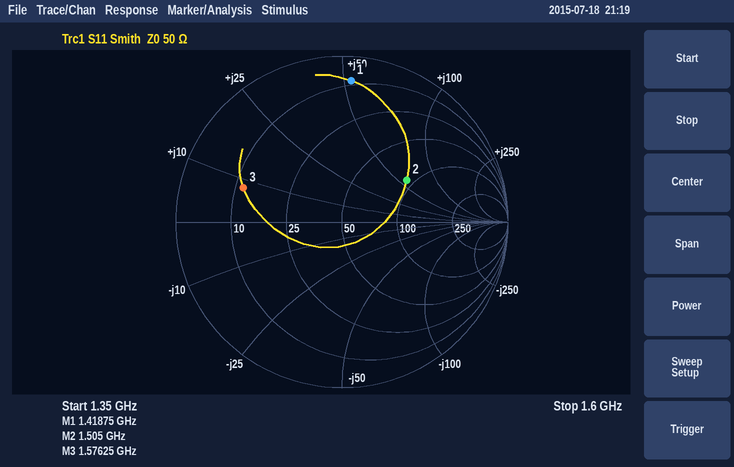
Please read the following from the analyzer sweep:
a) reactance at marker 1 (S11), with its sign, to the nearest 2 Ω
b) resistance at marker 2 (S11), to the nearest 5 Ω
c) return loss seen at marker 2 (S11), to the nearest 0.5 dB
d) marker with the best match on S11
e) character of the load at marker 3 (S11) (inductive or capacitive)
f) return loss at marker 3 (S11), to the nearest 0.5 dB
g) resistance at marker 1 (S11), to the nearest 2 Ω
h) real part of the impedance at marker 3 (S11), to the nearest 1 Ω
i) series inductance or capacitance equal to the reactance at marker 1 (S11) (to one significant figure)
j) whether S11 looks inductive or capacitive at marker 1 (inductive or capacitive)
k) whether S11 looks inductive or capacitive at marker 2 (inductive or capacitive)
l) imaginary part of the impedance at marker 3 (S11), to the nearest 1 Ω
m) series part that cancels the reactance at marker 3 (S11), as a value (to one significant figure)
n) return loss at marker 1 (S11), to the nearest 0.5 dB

+52 Ω
90 Ω
6.5 dB
marker 2
inductive
4.0 dB
8 Ω
12 Ω
6 nH
inductive
inductive
+8 Ω
10 pF
1.5 dB
